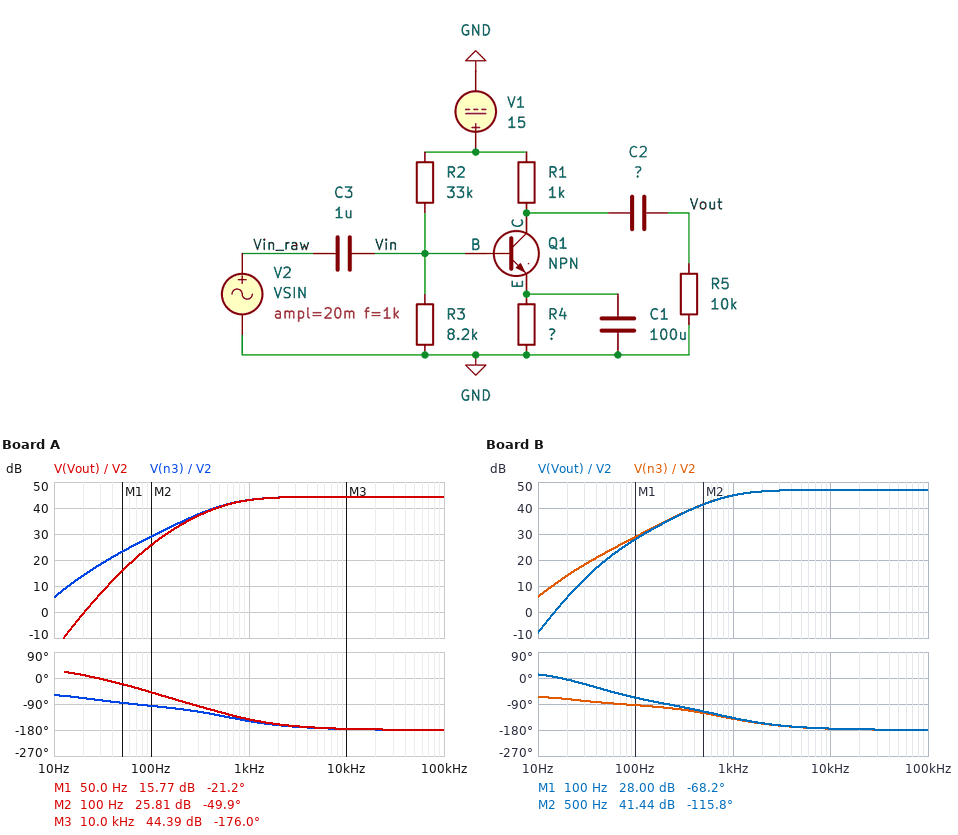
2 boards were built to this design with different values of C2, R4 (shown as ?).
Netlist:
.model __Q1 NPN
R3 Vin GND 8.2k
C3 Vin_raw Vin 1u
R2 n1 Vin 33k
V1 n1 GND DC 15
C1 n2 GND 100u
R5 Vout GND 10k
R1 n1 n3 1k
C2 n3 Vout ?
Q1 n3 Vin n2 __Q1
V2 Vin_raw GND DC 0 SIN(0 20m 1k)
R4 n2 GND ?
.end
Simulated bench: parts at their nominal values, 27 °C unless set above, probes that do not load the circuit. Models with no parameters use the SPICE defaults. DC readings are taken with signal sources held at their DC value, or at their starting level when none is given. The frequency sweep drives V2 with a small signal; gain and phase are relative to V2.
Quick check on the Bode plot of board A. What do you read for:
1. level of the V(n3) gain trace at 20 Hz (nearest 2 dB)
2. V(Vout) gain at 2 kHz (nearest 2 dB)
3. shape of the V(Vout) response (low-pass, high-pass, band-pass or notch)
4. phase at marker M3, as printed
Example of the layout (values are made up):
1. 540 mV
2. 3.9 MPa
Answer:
1. 14 dB
2. 44 dB
3. high-pass
4. -176.0 deg
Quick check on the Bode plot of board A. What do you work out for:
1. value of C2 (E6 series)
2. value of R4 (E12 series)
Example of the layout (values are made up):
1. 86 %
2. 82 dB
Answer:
1. 150 nF
2. 390 Ω
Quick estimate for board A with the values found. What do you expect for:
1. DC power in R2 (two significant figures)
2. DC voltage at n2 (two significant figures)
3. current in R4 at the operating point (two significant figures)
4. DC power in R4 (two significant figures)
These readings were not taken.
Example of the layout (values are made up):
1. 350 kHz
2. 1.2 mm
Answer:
1. 4.6 mW
2. 1.9 V
3. 4.8 mA
4. 8.9 mW
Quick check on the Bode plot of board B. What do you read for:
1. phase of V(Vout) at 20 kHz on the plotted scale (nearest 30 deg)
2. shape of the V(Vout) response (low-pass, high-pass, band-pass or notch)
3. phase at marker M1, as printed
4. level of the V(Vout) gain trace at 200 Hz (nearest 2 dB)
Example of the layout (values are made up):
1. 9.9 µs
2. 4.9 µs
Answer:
1. -180 deg
2. high-pass
3. -68.2 deg
4. 34 dB
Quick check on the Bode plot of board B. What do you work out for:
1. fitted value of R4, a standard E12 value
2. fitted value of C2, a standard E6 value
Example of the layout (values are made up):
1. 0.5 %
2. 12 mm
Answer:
1. 270 Ω
2. 330 nF
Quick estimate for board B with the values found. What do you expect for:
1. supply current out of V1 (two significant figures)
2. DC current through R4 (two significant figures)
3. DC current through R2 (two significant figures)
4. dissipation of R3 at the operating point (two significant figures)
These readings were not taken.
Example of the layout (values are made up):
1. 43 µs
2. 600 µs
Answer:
1. 6.8 mA
2. 6.5 mA
3. 380 µA
4. 800 µW
